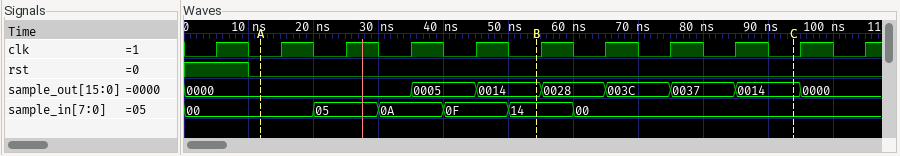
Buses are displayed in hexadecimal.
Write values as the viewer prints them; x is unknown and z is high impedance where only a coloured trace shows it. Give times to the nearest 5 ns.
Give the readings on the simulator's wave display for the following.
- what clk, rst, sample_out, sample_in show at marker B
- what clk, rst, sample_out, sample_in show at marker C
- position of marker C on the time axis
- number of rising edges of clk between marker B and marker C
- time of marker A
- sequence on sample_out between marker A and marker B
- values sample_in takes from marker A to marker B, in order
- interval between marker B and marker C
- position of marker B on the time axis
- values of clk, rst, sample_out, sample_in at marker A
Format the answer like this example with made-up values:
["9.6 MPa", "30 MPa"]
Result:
["clk=0, rst=0, sample_out=0014, sample_in=14", "clk=0, rst=0, sample_out=0014, sample_in=00", "95 ns", "4", "10 ns", "0000, 0005, 0014", "00, 05, 0A, 0F, 14", "40 ns", "55 ns", "clk=0, rst=0, sample_out=0000, sample_in=00"]
